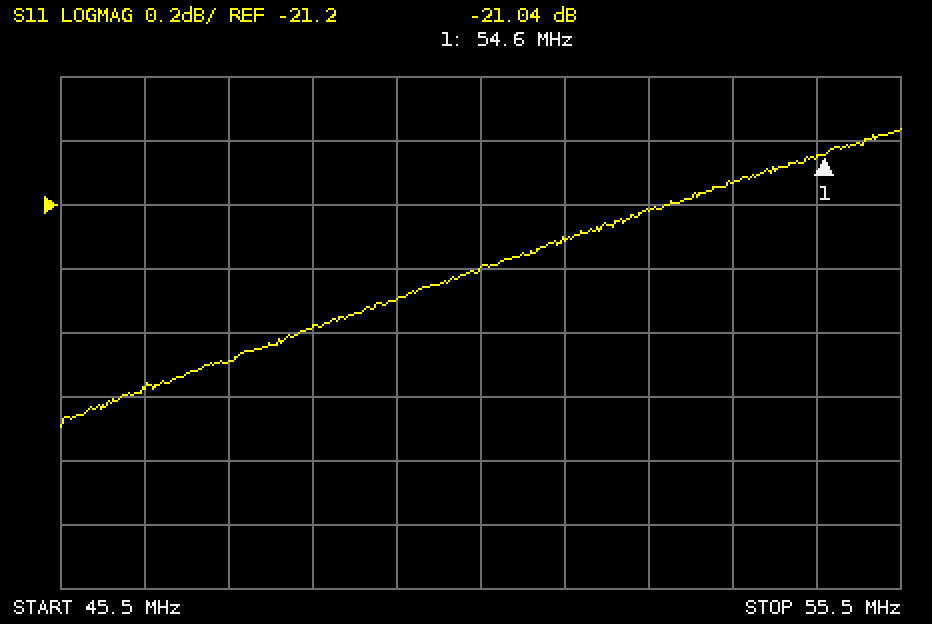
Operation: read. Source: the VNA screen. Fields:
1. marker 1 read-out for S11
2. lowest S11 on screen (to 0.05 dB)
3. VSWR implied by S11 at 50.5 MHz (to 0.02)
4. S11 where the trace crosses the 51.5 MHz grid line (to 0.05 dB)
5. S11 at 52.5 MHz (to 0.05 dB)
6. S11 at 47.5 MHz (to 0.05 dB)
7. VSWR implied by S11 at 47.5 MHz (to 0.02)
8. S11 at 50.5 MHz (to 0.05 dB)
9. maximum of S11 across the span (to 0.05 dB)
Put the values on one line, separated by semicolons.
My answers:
-21.04 dB; -21.90 dB; 1.18; -21.30 dB; -21.20 dB; -21.70 dB; 1.18; -21.40 dB; -20.95 dB
